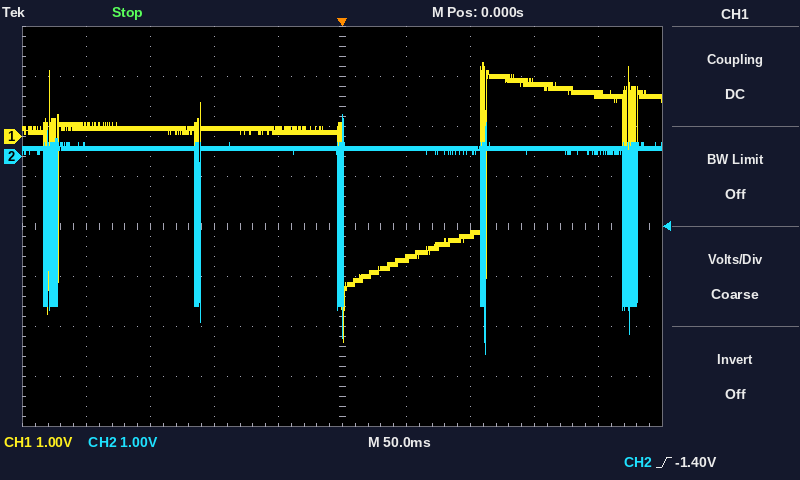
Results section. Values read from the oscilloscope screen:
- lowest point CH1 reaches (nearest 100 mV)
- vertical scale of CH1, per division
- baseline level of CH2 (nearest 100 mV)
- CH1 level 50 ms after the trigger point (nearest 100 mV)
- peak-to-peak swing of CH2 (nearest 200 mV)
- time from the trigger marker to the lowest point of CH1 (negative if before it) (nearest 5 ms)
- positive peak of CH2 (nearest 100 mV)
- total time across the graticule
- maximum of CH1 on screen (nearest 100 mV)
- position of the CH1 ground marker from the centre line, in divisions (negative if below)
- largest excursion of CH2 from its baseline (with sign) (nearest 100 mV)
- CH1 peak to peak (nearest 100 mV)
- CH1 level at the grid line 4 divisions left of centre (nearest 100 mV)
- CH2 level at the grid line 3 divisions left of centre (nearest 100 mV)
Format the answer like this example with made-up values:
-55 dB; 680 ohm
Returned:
-4.1 V; 1 V; 200 mV; -2.4 V; 4.8 V; 0 ms; 800 mV; 500 ms; 1.5 V; +1.8 div; -4.1 V; 5.6 V; 200 mV; 200 mV
